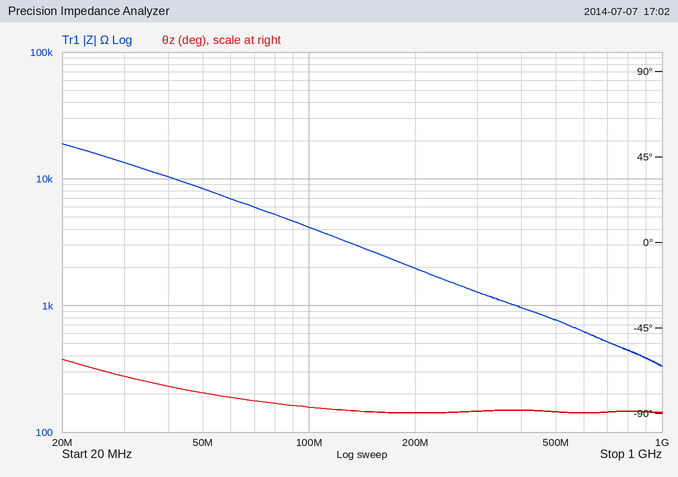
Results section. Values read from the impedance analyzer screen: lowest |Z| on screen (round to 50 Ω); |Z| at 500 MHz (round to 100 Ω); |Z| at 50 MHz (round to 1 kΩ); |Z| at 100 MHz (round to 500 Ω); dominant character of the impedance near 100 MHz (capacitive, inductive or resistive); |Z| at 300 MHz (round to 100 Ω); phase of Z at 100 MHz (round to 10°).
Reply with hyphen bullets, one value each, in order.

- 350 Ω
- 800 Ω
- 8 kΩ
- 4.0 kΩ
- capacitive
- 1.3 kΩ
- -90°
